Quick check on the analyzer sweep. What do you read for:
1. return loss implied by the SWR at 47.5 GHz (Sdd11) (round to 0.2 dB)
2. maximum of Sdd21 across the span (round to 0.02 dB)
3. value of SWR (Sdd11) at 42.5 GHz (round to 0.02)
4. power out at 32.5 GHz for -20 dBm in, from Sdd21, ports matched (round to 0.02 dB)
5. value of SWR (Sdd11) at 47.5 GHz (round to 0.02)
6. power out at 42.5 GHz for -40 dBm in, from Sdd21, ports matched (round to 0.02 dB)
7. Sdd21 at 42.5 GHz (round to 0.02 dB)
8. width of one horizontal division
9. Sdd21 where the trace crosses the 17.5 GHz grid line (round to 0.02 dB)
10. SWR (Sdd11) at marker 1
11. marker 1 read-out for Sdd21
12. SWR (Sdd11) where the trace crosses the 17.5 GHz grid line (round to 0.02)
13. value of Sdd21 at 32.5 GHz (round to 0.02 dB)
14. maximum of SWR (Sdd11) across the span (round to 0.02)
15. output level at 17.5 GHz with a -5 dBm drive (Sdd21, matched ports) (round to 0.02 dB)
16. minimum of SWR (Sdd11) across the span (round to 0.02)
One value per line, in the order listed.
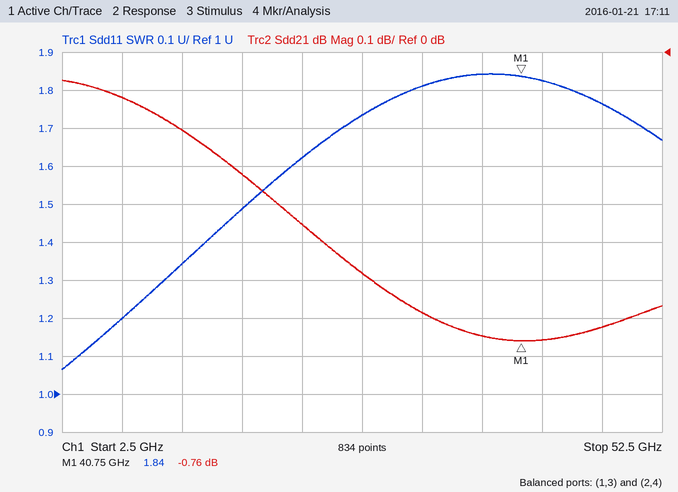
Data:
11.2 dB
-0.08 dB
1.82
-20.68 dBm
1.76
-40.76 dBm
-0.76 dB
5 GHz
-0.32 dB
1.84
-0.76 dB
1.48
-0.68 dB
1.84
-5.32 dBm
1.06
